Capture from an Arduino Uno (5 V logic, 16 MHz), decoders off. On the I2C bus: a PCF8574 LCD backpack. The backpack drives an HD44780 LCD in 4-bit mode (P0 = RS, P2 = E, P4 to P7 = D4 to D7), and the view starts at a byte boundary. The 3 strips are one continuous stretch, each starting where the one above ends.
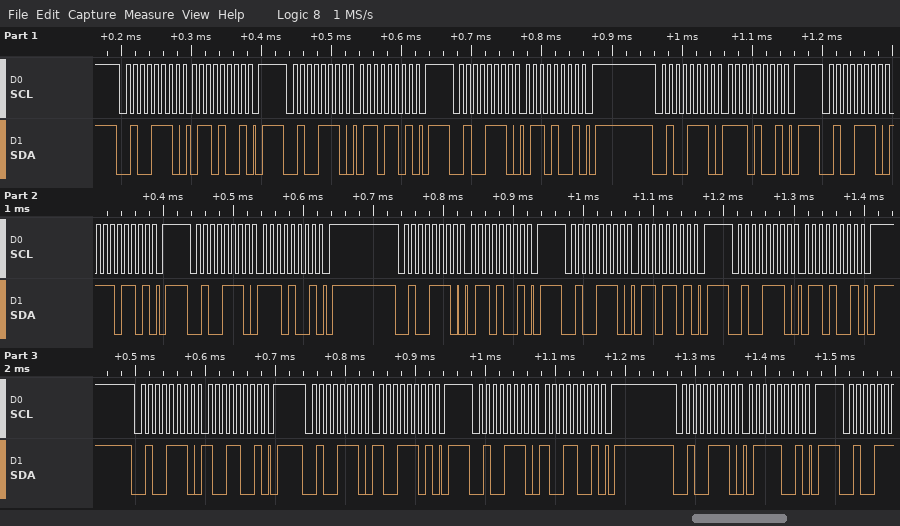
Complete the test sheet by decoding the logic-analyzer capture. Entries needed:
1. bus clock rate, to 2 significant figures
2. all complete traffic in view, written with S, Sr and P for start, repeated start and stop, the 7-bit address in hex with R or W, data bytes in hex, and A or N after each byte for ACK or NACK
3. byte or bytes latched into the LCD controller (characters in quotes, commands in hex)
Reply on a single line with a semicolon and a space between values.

100 kHz; S 27W A 69 A P S 27W A 6D A P S 27W A 69 A P S 27W A E9 A P S 27W A ED A P S 27W A E9 A P S 27W A 69 A P S 27W A 6D A P S 27W A 69 A P S 27W A 99 A P S 27W A 9D A P S 27W A 99 A P S 27W A 79 A P; 'n' 'i'
